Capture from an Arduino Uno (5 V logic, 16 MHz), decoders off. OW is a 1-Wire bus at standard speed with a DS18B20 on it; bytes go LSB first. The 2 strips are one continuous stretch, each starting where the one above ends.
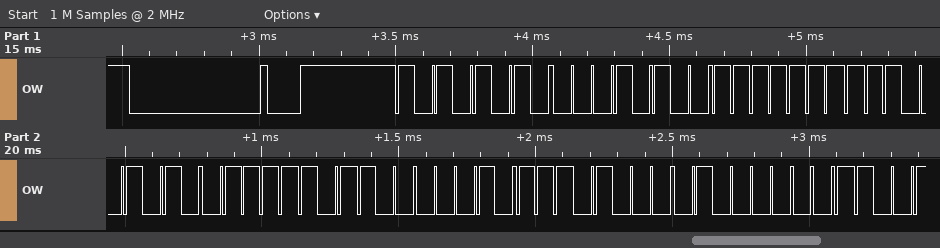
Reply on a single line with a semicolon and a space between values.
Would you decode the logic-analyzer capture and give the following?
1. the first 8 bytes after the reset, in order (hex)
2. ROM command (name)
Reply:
55 28 FF 53 BE 41 17 02; Match ROM
